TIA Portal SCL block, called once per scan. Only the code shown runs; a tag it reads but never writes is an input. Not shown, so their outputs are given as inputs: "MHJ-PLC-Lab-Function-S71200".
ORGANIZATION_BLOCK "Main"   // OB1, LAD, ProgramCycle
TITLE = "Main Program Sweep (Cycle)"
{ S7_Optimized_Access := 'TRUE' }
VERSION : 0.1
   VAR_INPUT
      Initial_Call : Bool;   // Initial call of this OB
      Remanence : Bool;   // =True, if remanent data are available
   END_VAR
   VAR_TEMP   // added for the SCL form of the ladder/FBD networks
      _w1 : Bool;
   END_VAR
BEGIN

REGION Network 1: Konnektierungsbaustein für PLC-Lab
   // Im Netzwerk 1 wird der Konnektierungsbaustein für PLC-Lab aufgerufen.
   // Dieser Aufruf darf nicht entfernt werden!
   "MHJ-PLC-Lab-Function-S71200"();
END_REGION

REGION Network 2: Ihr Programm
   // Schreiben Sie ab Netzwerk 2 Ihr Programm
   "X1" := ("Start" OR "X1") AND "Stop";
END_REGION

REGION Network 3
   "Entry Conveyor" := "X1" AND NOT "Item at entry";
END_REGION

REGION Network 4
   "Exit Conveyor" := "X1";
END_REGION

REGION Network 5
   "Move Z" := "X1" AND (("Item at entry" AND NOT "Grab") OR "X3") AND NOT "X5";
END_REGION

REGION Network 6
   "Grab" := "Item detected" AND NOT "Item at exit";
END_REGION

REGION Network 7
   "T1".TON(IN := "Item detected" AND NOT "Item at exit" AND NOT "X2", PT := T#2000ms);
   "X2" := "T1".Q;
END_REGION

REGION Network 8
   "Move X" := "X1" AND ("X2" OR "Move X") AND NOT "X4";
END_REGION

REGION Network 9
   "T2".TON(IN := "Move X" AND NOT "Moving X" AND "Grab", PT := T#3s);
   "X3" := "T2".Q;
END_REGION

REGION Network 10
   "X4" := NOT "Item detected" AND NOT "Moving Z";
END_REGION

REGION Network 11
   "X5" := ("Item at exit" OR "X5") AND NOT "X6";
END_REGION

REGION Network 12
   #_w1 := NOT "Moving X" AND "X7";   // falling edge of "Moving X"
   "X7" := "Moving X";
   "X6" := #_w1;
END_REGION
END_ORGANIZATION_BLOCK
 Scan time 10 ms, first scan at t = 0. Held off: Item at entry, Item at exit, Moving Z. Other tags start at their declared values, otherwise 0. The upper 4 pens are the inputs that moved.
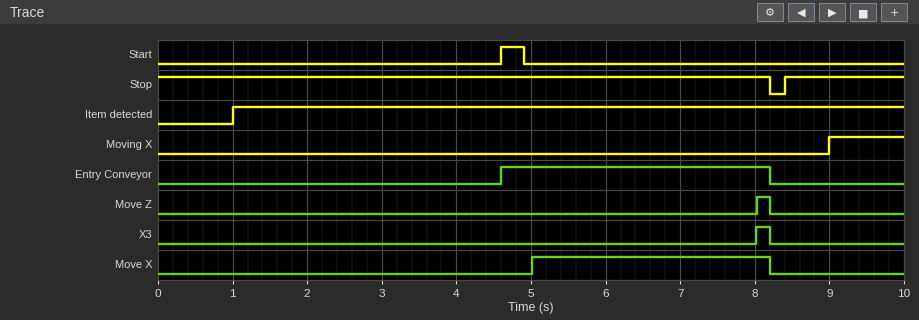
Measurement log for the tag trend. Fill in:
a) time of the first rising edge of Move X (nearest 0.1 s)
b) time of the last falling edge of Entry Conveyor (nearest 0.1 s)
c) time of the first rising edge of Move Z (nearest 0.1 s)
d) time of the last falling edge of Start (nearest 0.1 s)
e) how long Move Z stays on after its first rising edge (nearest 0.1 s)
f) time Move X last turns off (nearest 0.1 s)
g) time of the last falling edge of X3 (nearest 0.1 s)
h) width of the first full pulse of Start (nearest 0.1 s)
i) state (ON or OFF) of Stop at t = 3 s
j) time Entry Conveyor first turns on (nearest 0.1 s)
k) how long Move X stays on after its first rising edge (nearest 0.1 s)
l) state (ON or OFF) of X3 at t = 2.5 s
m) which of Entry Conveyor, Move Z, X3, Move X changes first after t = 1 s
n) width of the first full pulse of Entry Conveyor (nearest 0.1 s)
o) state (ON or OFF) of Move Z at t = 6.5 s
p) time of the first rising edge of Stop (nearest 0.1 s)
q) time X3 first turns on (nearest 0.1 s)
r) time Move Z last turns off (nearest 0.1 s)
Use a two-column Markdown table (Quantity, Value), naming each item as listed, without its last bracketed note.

| Quantity | Value |
|---|---|
| time of the first rising edge of Move X | 5.0 s |
| time of the last falling edge of Entry Conveyor | 8.2 s |
| time of the first rising edge of Move Z | 8.0 s |
| time of the last falling edge of Start | 4.9 s |
| how long Move Z stays on after its first rising edge | 0.2 s |
| time Move X last turns off | 8.2 s |
| time of the last falling edge of X3 | 8.2 s |
| width of the first full pulse of Start | 0.3 s |
| state (ON or OFF) of Stop at t = 3 s | ON |
| time Entry Conveyor first turns on | 4.6 s |
| how long Move X stays on after its first rising edge | 3.2 s |
| state (ON or OFF) of X3 at t = 2.5 s | OFF |
| which of Entry Conveyor, Move Z, X3, Move X changes first after t = 1 s | Entry Conveyor |
| width of the first full pulse of Entry Conveyor | 3.6 s |
| state (ON or OFF) of Move Z at t = 6.5 s | OFF |
| time of the first rising edge of Stop | 8.4 s |
| time X3 first turns on | 8.0 s |
| time Move Z last turns off | 8.2 s |
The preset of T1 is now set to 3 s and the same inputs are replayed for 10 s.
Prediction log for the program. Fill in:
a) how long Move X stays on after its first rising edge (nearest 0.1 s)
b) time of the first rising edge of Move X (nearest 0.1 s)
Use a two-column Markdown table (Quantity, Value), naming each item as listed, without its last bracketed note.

| Quantity | Value |
|---|---|
| how long Move X stays on after its first rising edge | 1.2 s |
| time of the first rising edge of Move X | 7.0 s |
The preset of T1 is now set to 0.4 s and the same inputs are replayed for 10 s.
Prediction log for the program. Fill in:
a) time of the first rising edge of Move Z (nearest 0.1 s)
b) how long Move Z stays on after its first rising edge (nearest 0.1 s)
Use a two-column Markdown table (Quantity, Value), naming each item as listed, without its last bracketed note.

| Quantity | Value |
|---|---|
| time of the first rising edge of Move Z | 7.8 s |
| how long Move Z stays on after its first rising edge | 0.4 s |
